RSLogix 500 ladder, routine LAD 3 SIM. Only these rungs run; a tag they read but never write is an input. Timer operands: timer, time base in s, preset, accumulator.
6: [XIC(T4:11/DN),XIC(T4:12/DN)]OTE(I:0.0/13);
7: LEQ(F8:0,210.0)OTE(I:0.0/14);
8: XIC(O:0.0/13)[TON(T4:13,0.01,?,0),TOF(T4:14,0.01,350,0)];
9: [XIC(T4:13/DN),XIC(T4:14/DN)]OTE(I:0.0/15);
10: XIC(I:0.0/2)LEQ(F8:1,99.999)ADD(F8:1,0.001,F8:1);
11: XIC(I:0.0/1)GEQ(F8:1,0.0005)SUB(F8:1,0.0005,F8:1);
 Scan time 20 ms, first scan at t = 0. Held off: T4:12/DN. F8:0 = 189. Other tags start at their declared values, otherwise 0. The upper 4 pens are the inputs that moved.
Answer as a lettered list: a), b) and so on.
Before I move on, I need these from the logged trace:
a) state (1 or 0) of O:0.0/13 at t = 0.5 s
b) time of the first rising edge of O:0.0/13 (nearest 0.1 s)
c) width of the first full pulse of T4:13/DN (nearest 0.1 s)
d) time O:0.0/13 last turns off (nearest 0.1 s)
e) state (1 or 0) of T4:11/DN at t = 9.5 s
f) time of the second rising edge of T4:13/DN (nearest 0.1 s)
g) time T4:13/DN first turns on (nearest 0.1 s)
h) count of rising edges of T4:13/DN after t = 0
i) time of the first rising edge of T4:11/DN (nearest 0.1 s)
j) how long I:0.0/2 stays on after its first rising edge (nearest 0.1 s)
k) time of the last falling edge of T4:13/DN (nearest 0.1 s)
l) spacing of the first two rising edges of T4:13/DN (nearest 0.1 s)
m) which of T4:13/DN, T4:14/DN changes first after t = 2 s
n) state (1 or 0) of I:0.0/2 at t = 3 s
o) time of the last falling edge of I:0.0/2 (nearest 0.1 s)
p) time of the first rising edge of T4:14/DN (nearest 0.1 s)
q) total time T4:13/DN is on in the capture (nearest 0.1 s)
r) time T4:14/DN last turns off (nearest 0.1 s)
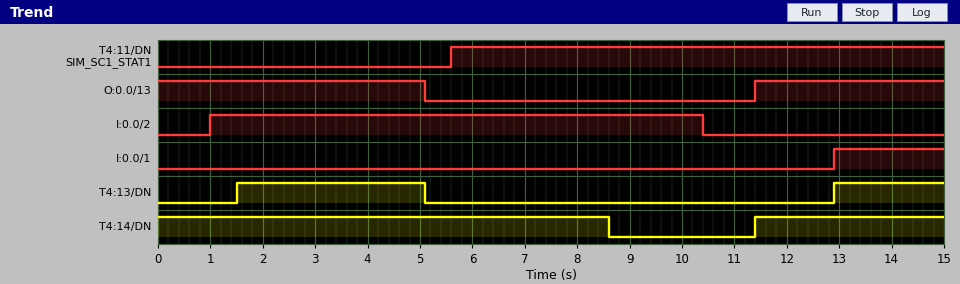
a) 1
b) 11.4 s
c) 3.6 s
d) 5.1 s
e) 1
f) 12.9 s
g) 1.5 s
h) 2
i) 5.6 s
j) 9.4 s
k) 5.1 s
l) 11.4 s
m) T4:13/DN
n) 1
o) 10.4 s
p) 11.4 s
q) 5.7 s
r) 8.6 s
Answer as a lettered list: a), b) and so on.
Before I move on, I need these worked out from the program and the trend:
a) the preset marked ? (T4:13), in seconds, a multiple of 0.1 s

a) 1.5 s
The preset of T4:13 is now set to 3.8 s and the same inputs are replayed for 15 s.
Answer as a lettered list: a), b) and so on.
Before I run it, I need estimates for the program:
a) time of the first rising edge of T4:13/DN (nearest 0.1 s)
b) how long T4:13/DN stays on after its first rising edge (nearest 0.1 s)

a) 3.8 s
b) 1.3 s
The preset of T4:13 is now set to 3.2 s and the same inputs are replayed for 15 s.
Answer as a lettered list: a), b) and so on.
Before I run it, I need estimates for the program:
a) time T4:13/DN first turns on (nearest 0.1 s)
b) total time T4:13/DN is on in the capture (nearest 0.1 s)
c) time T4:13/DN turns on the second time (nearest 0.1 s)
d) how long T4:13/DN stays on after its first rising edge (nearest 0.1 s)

a) 3.2 s
b) 2.3 s
c) 14.6 s
d) 1.9 s
